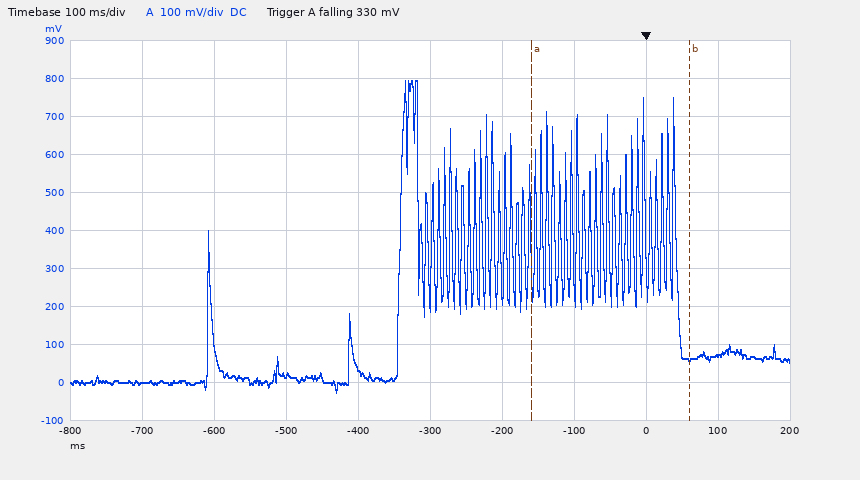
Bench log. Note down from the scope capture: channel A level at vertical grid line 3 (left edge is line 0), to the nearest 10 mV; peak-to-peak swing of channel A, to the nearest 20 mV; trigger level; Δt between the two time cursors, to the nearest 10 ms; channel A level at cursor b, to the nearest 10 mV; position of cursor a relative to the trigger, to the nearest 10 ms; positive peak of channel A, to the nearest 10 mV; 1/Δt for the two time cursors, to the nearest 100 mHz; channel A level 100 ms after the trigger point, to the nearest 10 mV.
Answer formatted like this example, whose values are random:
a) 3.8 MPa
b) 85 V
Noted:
a) 20 mV
b) 820 mV
c) 330 mV
d) 220 ms
e) 60 mV
f) -160 ms
g) 790 mV
h) 4.5 Hz
i) 70 mV
